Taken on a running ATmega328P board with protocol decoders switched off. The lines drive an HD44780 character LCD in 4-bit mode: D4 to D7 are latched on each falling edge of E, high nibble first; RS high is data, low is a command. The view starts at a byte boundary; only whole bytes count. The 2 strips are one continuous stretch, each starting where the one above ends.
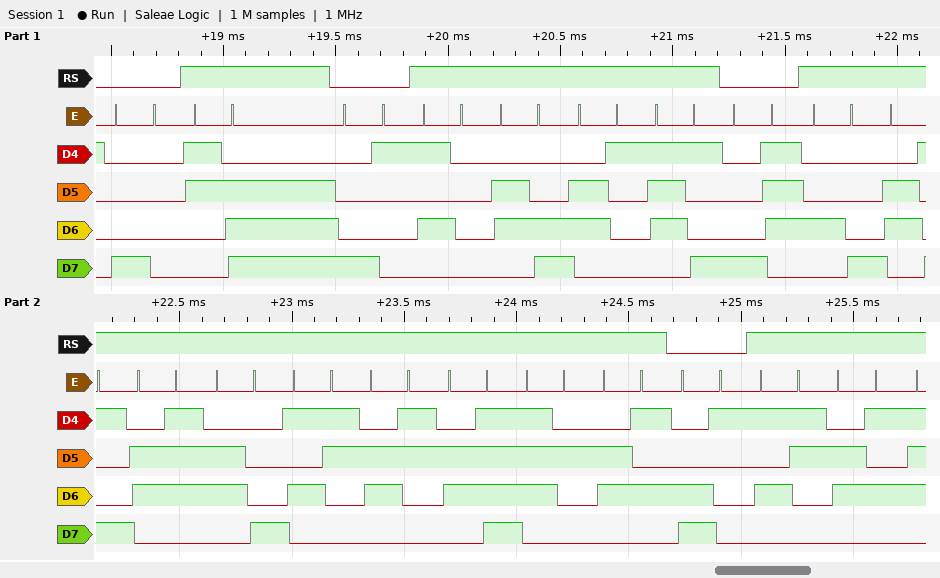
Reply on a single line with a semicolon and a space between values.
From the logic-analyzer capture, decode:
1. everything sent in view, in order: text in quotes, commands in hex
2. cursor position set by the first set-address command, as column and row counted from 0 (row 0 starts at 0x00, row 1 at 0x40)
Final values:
0x80 ">" 0x81 "Play" 0x87 "HighScore" 0xC1 "Se"; column 0, row 0
